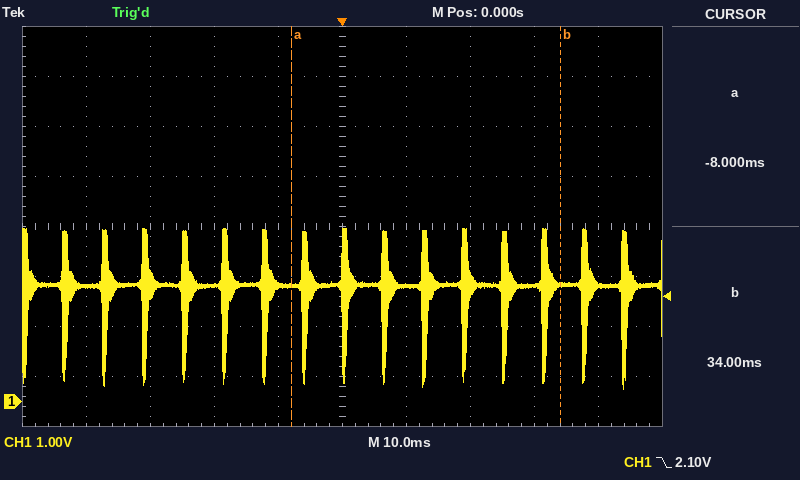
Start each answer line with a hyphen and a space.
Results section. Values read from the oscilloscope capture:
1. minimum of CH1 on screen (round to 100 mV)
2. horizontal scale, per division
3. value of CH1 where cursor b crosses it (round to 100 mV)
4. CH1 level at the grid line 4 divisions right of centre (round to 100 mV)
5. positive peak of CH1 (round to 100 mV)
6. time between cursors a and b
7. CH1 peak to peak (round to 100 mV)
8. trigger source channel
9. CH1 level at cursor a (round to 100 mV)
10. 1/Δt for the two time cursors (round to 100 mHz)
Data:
- 300 mV
- 10 ms
- 2.3 V
- 2.3 V
- 3.5 V
- 42 ms
- 3.2 V
- CH1
- 2.3 V
- 23.8 Hz
